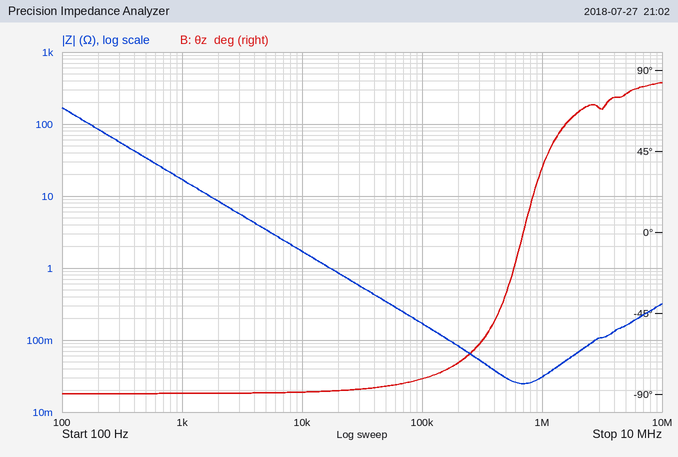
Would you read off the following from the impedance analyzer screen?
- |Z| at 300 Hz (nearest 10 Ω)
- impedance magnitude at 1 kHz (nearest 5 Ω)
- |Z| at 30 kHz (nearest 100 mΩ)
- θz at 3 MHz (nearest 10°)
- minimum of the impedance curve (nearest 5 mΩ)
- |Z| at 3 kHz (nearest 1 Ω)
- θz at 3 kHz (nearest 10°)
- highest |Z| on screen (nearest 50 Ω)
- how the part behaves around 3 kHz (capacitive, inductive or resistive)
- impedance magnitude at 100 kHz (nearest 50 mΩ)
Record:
60 Ω
15 Ω
600 mΩ
70°
25 mΩ
6 Ω
-90°
150 Ω
capacitive
150 mΩ
